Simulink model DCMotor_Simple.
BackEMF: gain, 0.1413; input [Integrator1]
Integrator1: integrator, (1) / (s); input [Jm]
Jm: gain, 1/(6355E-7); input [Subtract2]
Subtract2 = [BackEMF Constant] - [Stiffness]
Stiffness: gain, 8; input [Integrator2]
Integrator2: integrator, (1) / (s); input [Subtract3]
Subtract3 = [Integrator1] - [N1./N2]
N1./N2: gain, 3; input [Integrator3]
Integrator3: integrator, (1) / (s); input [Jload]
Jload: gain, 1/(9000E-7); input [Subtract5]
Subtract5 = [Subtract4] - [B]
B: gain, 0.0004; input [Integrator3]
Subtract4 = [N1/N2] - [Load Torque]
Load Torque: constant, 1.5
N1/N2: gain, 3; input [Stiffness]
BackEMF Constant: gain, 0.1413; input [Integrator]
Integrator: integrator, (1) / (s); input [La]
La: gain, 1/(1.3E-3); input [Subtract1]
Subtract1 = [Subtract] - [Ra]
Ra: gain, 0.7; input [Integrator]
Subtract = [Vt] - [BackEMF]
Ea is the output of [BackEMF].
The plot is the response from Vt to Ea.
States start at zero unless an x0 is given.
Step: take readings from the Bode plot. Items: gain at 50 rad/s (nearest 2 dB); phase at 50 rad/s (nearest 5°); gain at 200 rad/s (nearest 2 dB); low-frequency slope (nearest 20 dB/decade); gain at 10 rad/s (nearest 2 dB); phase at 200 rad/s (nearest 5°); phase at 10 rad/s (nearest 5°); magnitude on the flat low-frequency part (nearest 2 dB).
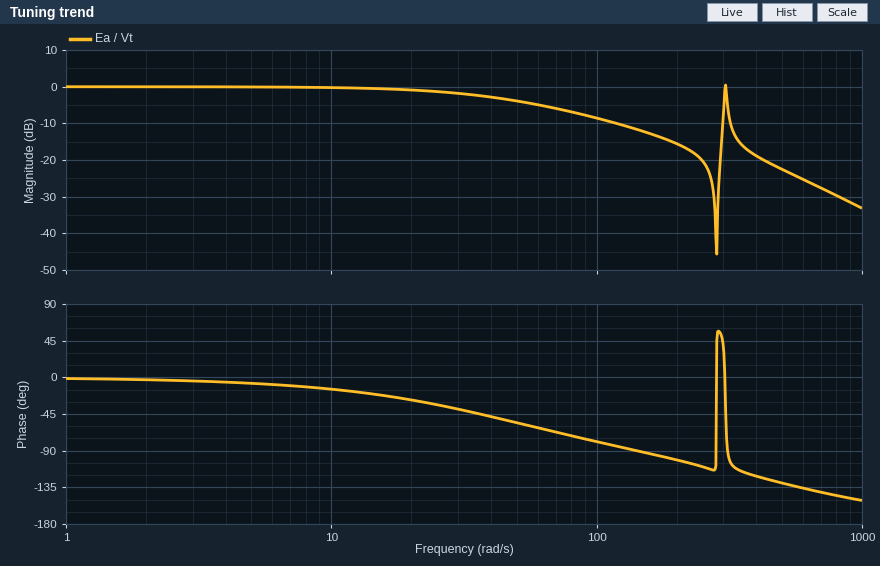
-4 dB
-55°
-16 dB
0 dB/decade
0 dB
-100°
-15°
0 dB
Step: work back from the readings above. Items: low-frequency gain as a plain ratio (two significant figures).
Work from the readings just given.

1.0
